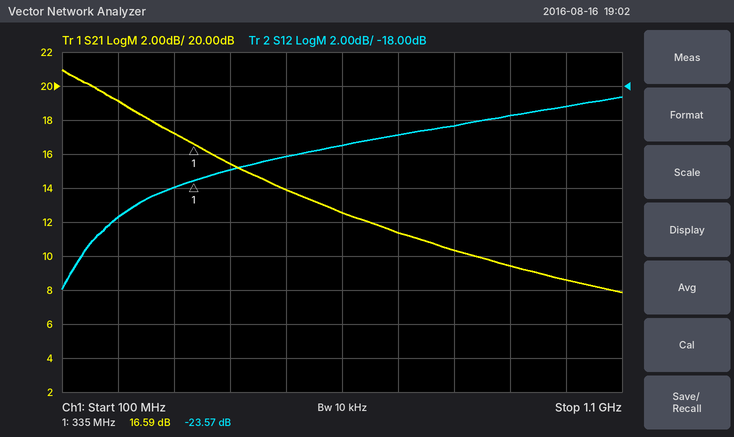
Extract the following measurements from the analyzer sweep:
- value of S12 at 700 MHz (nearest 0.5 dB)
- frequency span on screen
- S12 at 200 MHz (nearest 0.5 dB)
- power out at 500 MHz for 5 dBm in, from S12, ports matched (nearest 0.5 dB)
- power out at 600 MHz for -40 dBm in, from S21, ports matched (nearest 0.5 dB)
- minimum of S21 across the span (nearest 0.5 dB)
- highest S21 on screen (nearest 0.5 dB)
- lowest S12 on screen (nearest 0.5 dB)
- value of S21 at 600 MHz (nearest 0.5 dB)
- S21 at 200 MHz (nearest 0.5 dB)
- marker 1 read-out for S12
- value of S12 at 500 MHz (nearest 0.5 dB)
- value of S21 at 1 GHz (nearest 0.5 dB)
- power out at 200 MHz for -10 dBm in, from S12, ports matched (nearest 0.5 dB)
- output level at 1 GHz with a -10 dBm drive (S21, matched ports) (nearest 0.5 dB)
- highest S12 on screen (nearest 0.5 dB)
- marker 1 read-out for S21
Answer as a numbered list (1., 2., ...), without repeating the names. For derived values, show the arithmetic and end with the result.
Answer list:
1. -21.0 dB
2. 1 GHz
3. -25.5 dB
4. 5 dBm + (-22.0 dB) = -17.0 dBm
5. -40 dBm + (12.5 dB) = -27.5 dBm
6. 8.0 dB
7. 21.0 dB
8. -30.0 dB
9. 12.5 dB
10. 19.0 dB
11. -23.57 dB
12. -22.0 dB
13. 8.5 dB
14. -10 dBm + (-25.5 dB) = -35.5 dBm
15. -10 dBm + (8.5 dB) = -1.5 dBm
16. -18.5 dB
17. 16.59 dB
